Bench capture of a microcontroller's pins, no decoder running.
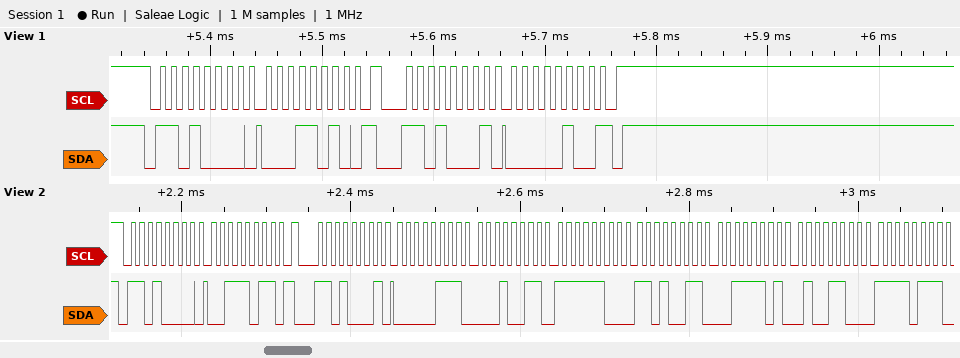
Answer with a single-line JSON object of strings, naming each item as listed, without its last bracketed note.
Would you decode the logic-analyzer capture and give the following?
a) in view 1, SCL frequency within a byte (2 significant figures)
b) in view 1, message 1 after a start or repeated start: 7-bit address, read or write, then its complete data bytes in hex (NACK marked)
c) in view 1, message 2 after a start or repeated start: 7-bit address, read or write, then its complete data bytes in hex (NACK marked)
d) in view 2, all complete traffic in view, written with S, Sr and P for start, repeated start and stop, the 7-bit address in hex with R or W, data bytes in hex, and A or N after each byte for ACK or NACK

{"in view 1, SCL frequency within a byte": "100 kHz", "in view 1, message 1 after a start or repeated start: 7-bit address, read or write, then its complete data bytes in hex": "0x68 write: 1A", "in view 1, message 2 after a start or repeated start: 7-bit address, read or write, then its complete data bytes in hex": "0x68 read: 04 NACK", "in view 2, all complete traffic in view, written with S, Sr and P for start, repeated start and stop, the 7-bit address in hex with R or W, data bytes in hex, and A or N after each byte for ACK or NACK": "S 68W A 3B A Sr 68R A 07 A 13 A FC A D3 A 3D A 4C A F7 A"}
